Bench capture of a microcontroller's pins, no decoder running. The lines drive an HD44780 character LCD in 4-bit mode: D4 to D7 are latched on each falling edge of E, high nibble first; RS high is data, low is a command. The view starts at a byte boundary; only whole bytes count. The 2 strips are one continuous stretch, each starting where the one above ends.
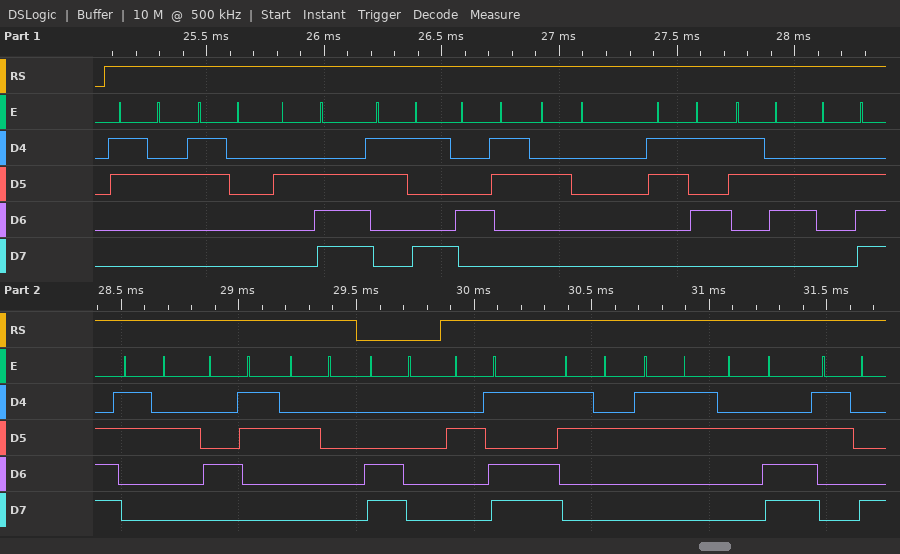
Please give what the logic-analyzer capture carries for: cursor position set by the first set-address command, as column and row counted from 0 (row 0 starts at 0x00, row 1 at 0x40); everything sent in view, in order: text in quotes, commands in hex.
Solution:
column 0, row 1
"20.9C 56.2C " 0xC0 "-23.8"
